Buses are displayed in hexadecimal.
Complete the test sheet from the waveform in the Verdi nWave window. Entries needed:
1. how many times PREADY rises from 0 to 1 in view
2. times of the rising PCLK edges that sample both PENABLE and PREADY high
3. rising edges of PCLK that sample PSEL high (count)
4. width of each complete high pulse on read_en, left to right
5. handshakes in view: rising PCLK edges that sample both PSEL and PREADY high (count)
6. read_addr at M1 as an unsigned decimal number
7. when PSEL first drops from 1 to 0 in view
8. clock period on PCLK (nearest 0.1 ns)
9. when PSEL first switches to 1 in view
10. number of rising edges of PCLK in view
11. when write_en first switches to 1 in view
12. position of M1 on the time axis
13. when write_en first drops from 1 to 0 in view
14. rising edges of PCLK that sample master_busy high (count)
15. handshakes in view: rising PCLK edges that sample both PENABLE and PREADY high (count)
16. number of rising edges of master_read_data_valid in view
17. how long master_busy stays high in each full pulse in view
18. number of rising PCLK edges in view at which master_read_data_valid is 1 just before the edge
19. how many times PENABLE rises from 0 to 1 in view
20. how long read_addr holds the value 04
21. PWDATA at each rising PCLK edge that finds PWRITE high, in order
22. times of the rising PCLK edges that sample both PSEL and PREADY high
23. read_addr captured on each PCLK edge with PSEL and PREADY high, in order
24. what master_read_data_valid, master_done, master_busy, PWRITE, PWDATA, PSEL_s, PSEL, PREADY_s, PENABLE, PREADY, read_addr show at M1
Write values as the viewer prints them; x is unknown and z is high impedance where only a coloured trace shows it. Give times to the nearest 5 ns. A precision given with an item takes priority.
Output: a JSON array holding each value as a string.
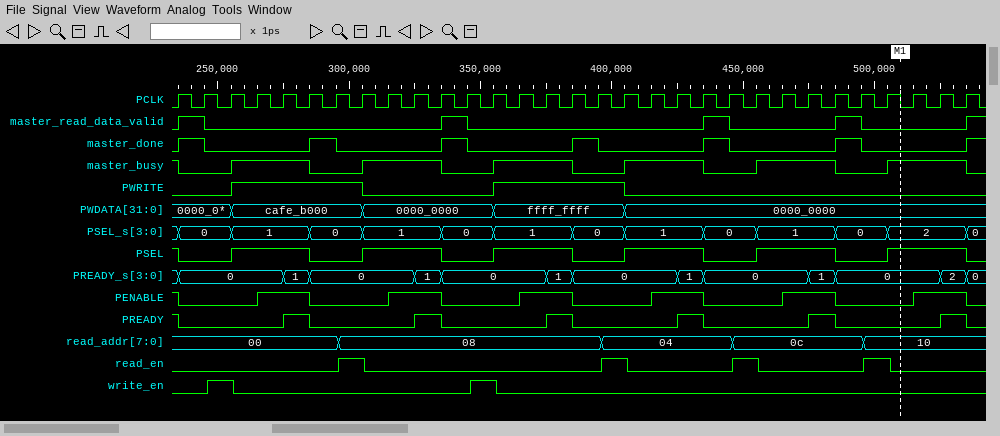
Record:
["6", "235 ns, 285 ns, 335 ns, 385 ns, 435 ns, 485 ns, 535 ns", "19", "10 ns, 10 ns, 10 ns, 10 ns", "7", "16", "235 ns", "10 ns", "255 ns", "31", "245 ns", "510 ns", "255 ns", "19", "7", "5", "30 ns, 30 ns, 30 ns, 30 ns, 30 ns, 30 ns", "4", "6", "50 ns", "cafe_b000, cafe_b000, cafe_b000, cafe_b000, cafe_b000, ffff_ffff, ffff_ffff, ffff_ffff, ffff_ffff, ffff_ffff", "235 ns, 285 ns, 335 ns, 385 ns, 435 ns, 485 ns, 535 ns", "00, 00, 08, 08, 04, 0c, 10", "master_read_data_valid=0, master_done=0, master_busy=1, PWRITE=0, PWDATA=0000_0000, PSEL_s=2, PSEL=1, PREADY_s=0, PENABLE=0, PREADY=0, read_addr=10"]
